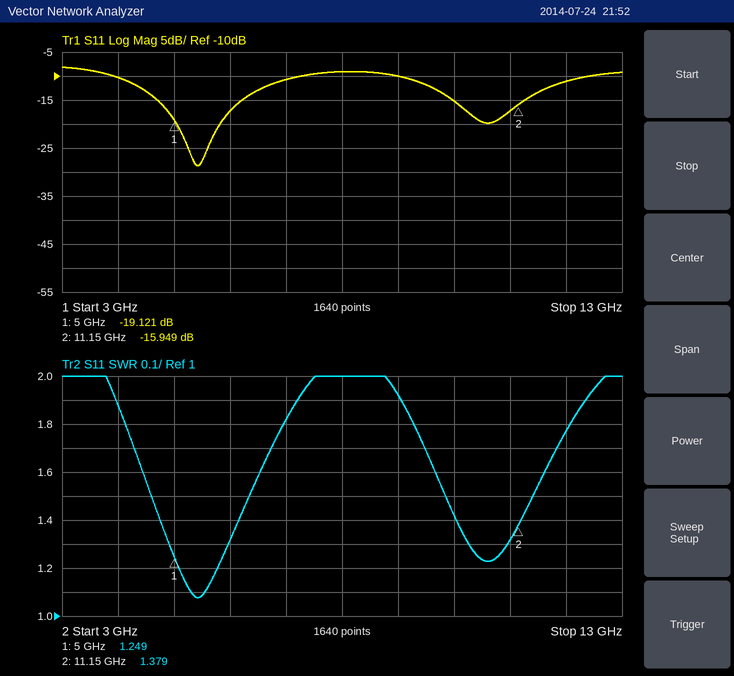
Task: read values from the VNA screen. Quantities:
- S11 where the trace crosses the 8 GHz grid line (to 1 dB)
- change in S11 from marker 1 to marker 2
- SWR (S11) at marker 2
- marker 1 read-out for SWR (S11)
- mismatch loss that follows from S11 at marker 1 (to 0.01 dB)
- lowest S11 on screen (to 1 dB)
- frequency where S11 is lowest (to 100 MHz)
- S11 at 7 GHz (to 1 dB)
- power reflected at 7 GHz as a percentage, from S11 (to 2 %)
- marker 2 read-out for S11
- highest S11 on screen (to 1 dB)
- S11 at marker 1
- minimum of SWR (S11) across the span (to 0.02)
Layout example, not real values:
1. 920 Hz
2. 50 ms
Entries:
1. -9 dB
2. 3.172 dB
3. 1.379
4. 1.249
5. 0.05 dB
6. -29 dB
7. 5.4 GHz
8. -11 dB
9. 8 %
10. -15.949 dB
11. -8 dB
12. -19.121 dB
13. 1.08
